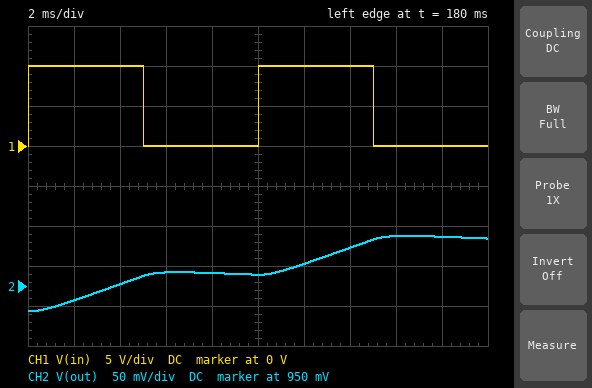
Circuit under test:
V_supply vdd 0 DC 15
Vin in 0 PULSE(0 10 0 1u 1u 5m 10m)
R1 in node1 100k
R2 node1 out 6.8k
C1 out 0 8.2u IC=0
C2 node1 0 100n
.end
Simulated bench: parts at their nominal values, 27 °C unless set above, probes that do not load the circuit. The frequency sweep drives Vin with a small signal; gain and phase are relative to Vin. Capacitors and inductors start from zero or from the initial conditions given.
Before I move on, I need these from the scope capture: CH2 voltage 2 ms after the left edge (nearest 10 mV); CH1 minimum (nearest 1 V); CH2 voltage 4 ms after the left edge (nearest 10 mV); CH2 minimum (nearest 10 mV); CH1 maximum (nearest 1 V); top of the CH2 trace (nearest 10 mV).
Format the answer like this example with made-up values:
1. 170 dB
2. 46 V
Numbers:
1. 930 mV
2. 0 V
3. 950 mV
4. 920 mV
5. 10 V
6. 1.01 V
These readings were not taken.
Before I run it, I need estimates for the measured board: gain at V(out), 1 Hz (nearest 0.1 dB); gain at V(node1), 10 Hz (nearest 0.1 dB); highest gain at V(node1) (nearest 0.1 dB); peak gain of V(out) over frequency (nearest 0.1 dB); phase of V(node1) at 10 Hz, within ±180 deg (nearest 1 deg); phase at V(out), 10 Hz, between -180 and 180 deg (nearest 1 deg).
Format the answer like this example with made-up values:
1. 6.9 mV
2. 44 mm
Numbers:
1. -15.0 dB
2. -23.7 dB
3. 0 dB
4. 0 dB
5. -17 deg
6. -91 deg
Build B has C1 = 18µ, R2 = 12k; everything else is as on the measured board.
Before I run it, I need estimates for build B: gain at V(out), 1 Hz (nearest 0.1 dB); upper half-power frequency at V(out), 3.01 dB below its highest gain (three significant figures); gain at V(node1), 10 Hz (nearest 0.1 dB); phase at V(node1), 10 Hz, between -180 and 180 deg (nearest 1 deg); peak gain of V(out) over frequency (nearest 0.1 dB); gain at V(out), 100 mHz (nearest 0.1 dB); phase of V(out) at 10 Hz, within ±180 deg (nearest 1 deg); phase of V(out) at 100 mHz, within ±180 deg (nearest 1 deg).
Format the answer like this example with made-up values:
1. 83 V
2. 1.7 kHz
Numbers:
1. -22.1 dB
2. 78.6 mHz
3. -19.4 dB
4. -8 deg
5. 0 dB
6. -4.2 dB
7. -93 deg
8. -52 deg
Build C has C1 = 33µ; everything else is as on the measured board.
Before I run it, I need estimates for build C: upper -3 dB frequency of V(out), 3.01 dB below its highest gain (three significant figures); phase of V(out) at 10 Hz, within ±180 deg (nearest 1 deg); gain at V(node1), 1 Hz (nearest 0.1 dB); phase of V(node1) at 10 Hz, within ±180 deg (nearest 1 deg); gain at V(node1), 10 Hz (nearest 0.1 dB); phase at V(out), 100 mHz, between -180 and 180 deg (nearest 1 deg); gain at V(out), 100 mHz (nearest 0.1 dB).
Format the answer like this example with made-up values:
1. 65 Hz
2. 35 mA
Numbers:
1. 45.0 mHz
2. -92 deg
3. -22.2 dB
4. -6 deg
5. -23.9 dB
6. -66 deg
7. -7.7 dB
